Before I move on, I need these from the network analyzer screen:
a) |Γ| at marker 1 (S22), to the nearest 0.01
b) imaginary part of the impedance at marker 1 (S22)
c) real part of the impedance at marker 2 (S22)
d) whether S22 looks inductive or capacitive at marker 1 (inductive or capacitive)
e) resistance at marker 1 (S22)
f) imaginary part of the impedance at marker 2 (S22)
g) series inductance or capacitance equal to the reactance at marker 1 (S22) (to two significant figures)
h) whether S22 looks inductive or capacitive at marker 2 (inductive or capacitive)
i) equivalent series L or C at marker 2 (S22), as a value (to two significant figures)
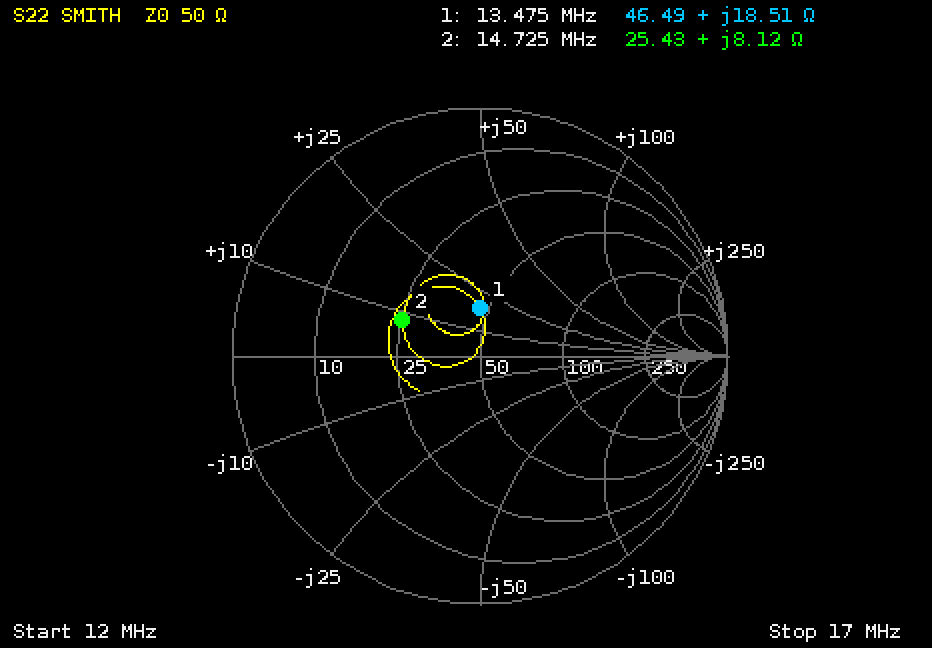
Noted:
0.19
+18.51 Ω
25.43 Ω
inductive
46.49 Ω
+8.12 Ω
220 nH
inductive
88 nH
